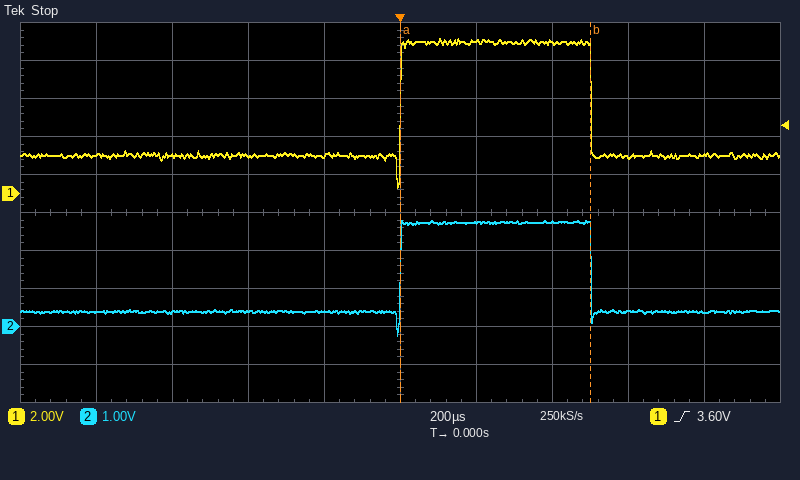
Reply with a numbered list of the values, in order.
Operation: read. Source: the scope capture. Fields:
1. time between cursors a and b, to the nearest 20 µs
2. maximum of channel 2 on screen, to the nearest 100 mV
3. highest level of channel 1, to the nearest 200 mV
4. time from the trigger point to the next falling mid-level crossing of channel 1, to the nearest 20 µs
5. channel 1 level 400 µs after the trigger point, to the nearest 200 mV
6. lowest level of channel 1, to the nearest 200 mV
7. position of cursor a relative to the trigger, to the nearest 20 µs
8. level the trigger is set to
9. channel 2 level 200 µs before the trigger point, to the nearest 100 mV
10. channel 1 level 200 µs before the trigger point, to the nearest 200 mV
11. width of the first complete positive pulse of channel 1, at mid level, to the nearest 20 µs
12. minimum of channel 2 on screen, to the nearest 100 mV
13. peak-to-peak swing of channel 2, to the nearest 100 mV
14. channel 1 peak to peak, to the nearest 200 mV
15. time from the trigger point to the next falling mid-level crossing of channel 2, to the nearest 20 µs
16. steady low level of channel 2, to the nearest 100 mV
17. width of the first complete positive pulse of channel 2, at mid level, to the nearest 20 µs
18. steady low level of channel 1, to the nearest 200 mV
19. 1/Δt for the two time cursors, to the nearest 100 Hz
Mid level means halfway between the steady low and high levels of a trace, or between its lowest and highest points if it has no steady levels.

1. 500 µs
2. 2.8 V
3. 8.2 V
4. 500 µs
5. 8.0 V
6. 400 mV
7. 0 µs
8. 3.60 V
9. 400 mV
10. 2.0 V
11. 500 µs
12. -200 mV
13. 3.0 V
14. 7.8 V
15. 500 µs
16. 400 mV
17. 500 µs
18. 2.0 V
19. 2.0 kHz
